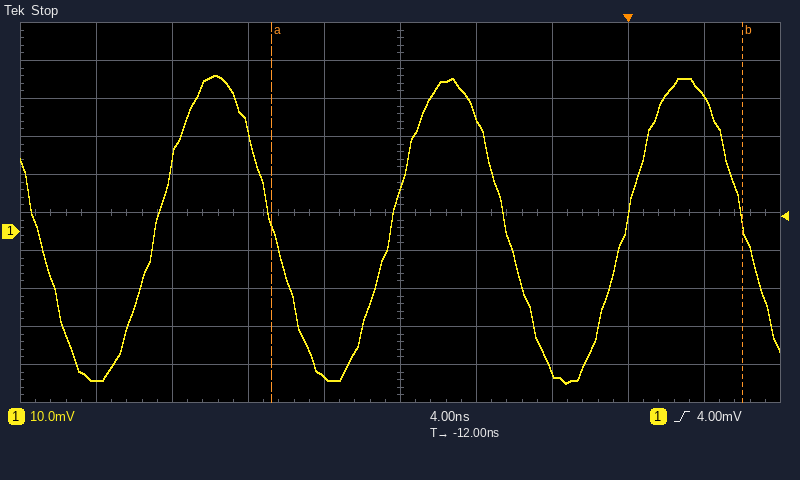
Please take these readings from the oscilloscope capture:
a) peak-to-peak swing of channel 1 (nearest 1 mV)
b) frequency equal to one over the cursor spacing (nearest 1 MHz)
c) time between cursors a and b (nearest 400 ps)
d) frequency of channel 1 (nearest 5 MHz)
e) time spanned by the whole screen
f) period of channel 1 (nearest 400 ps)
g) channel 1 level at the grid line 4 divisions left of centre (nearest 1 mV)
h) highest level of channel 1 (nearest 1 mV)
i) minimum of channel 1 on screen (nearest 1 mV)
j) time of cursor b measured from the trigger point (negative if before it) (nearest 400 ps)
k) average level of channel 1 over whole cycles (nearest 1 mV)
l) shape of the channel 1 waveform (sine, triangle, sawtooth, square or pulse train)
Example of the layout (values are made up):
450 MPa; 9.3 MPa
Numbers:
81 mV; 40 MHz; 24.8 ns; 80 MHz; 40 ns; 12.4 ns; -39 mV; 41 mV; -40 mV; +6.0 ns; 1 mV; sine
